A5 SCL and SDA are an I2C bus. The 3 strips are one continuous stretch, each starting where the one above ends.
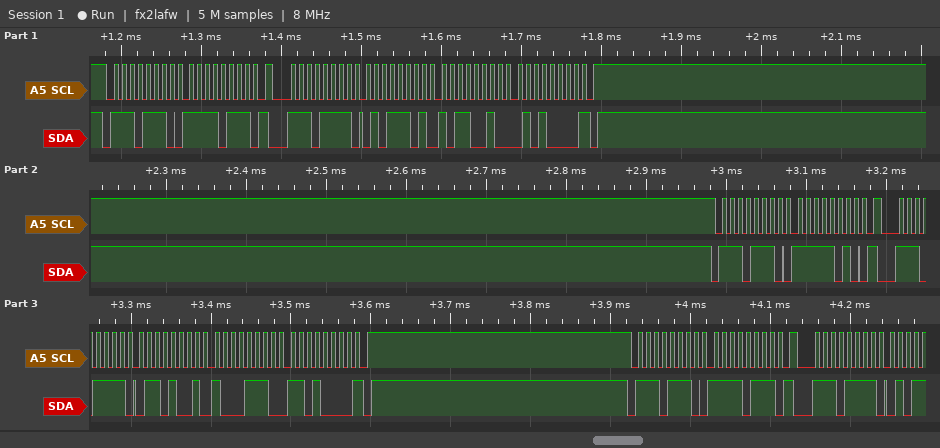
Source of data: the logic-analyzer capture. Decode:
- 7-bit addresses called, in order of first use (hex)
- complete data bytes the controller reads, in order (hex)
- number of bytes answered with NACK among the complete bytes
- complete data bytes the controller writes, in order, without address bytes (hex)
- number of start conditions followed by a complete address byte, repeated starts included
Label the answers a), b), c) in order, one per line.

a) 0x77
b) 5D B2 50 69 8E D0
c) 2
d) F7 FA F7
e) 6
